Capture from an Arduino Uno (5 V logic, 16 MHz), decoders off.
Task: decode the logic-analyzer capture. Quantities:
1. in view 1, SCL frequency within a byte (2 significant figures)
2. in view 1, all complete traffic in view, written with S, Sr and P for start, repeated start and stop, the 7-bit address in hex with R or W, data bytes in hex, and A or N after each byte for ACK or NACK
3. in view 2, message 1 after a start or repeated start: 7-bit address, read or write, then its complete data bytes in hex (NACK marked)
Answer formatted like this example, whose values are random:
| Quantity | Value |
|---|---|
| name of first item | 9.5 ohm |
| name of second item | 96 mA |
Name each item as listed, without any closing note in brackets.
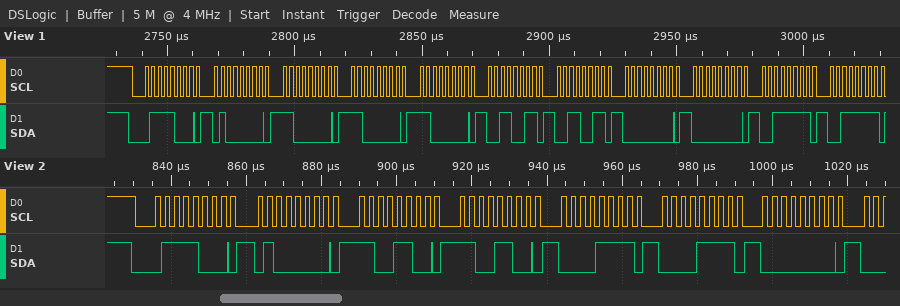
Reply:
| Quantity | Value |
|---|---|
| in view 1, SCL frequency within a byte | 400 kHz |
| in view 1, all complete traffic in view, written with S, Sr and P for start, repeated start and stop, the 7-bit address in hex with R or W, data bytes in hex, and A or N after each byte for ACK or NACK | S 3CW A 40 A C0 A C0 A C0 A 33 A 33 A 00 A 00 A 3F A 3F A |
| in view 2, message 1 after a start or repeated start: 7-bit address, read or write, then its complete data bytes in hex | 0x3C write: 40 CC CC 0F 0F 00 |
